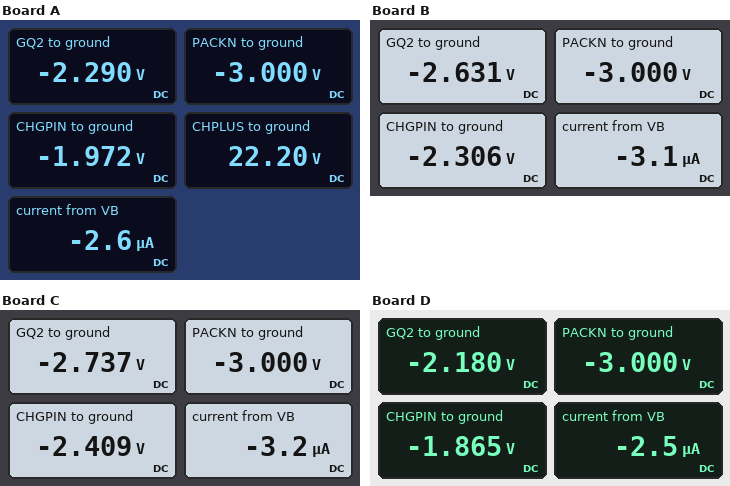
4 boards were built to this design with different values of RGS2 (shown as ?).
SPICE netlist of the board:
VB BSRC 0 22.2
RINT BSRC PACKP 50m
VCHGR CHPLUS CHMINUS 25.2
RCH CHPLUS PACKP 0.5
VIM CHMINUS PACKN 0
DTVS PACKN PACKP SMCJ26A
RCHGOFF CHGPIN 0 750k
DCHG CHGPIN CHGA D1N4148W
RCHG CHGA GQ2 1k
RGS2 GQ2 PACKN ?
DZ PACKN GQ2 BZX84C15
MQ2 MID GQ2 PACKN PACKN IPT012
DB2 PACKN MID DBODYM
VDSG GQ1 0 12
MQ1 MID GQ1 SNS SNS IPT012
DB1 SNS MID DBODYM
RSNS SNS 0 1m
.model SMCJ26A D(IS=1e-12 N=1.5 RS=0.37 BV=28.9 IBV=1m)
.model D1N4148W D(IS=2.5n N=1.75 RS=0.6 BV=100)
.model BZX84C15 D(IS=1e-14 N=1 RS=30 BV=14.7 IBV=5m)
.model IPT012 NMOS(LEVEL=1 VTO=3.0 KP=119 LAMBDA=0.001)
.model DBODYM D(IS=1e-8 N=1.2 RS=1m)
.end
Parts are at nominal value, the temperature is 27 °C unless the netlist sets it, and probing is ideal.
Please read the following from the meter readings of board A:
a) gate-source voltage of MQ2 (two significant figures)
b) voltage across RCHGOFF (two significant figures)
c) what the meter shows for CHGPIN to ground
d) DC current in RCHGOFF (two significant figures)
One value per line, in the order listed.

710 mV
2.0 V
-1.972 V
2.6 µA
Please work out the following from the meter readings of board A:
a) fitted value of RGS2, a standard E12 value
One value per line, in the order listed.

270 kΩ
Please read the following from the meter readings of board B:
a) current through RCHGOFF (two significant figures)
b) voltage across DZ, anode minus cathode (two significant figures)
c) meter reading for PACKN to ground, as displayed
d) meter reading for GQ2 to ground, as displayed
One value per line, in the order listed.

3.1 µA
-370 mV
-3.000 V
-2.631 V
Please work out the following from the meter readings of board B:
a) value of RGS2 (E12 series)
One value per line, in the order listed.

120 kΩ
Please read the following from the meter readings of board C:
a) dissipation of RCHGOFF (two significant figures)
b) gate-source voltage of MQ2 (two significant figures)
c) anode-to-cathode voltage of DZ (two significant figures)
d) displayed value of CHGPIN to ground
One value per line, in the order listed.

7.7 µW
260 mV
-260 mV
-2.409 V
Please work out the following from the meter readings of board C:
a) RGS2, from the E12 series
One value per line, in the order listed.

82 kΩ
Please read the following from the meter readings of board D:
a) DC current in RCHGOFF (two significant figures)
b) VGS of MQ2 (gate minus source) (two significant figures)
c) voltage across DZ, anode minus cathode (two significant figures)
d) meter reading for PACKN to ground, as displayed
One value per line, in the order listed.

2.5 µA
820 mV
-820 mV
-3.000 V
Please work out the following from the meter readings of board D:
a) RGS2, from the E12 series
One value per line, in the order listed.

330 kΩ
